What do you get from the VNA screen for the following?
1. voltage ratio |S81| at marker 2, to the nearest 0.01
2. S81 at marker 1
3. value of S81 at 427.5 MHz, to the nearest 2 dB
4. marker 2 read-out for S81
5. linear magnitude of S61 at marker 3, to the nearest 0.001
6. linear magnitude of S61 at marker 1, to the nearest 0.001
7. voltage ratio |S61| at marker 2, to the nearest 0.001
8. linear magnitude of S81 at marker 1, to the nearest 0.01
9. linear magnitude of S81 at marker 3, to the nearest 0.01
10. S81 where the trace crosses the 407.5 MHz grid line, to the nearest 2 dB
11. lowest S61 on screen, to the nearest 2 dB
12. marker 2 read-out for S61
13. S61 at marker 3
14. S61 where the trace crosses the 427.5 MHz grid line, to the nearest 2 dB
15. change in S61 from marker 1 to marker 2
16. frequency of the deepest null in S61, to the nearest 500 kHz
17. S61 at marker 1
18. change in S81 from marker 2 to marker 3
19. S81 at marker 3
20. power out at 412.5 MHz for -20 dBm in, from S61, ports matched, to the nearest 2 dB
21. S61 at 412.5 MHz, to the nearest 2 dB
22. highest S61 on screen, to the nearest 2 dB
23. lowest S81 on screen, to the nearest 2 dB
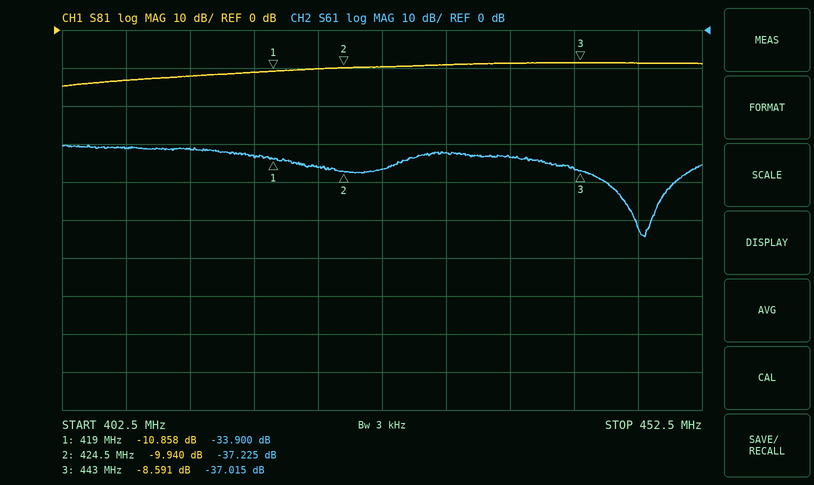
0.32
-10.858 dB
-10 dB
-9.940 dB
0.014
0.020
0.014
0.29
0.37
-14 dB
-54 dB
-37.225 dB
-37.015 dB
-36 dB
-3.325 dB
448.0 MHz
-33.900 dB
1.349 dB
-8.591 dB
-52 dBm
-32 dB
-30 dB
-14 dB
